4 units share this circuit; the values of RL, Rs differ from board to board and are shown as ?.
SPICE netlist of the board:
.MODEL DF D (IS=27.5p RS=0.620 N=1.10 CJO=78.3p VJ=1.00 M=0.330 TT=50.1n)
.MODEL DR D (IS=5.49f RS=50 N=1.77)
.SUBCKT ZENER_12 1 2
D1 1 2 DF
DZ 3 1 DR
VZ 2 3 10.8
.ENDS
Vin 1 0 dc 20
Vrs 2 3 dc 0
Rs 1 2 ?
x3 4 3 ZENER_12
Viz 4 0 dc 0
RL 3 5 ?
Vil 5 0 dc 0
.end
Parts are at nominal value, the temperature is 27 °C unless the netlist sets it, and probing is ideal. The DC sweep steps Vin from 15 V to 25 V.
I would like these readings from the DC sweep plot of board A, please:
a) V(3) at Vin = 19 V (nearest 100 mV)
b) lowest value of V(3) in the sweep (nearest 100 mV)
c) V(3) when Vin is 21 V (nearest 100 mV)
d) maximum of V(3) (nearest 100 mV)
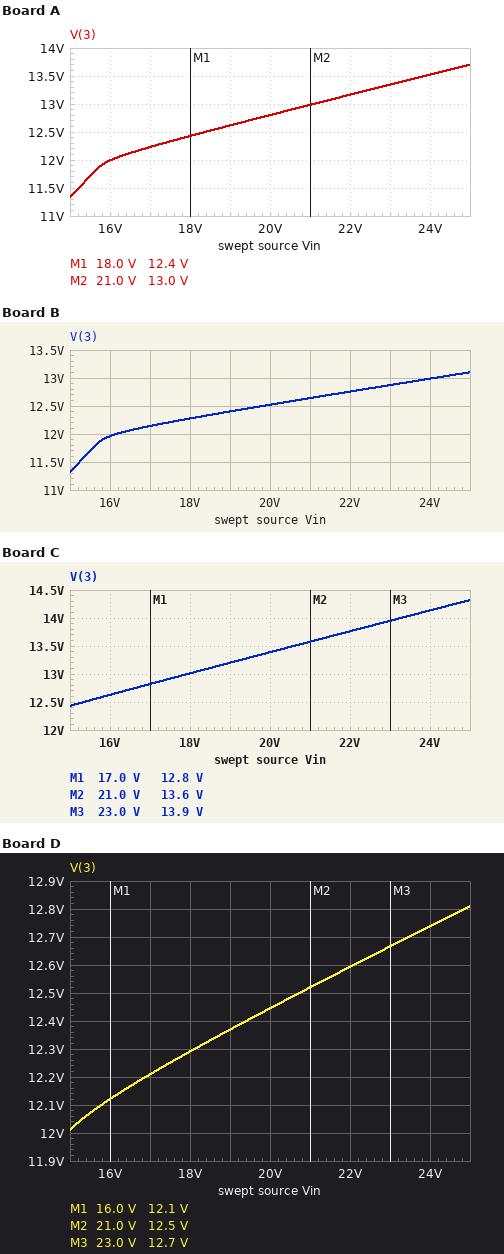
12.6 V
11.3 V
13.0 V
13.7 V
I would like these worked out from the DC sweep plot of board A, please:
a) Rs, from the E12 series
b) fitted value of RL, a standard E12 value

220 Ω
680 Ω
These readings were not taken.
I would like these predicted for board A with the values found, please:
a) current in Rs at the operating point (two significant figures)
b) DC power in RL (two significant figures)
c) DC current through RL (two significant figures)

33 mA
240 mW
19 mA
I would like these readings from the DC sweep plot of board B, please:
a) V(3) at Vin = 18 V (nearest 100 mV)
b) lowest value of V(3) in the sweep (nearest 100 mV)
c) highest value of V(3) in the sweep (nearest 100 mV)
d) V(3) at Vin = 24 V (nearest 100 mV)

12.3 V
11.3 V
13.1 V
13.0 V
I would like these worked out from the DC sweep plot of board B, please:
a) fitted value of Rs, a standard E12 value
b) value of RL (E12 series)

390 Ω
1.2 kΩ
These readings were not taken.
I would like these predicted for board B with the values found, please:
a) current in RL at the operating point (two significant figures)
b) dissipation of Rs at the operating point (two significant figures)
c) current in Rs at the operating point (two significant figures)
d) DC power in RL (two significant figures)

10 mA
140 mW
19 mA
130 mW
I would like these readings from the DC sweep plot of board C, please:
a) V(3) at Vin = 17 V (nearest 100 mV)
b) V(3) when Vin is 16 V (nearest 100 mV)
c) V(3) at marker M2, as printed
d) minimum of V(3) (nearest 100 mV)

12.8 V
12.6 V
13.6 V
12.4 V
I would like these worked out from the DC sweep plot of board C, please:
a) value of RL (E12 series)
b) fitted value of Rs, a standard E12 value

2.7 kΩ
220 Ω
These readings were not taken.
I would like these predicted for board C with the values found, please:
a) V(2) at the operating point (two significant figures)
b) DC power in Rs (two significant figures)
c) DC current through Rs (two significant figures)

13 V
200 mW
30 mA
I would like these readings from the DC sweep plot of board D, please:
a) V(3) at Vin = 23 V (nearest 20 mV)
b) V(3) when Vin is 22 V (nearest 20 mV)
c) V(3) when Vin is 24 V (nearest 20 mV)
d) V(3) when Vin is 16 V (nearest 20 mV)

12.66 V
12.60 V
12.74 V
12.12 V
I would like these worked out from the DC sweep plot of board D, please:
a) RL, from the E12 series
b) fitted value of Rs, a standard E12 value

3.3 kΩ
680 Ω
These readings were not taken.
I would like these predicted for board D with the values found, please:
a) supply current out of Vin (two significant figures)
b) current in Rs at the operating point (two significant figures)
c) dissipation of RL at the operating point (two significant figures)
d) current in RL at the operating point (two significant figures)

11 mA
11 mA
47 mW
3.8 mA
